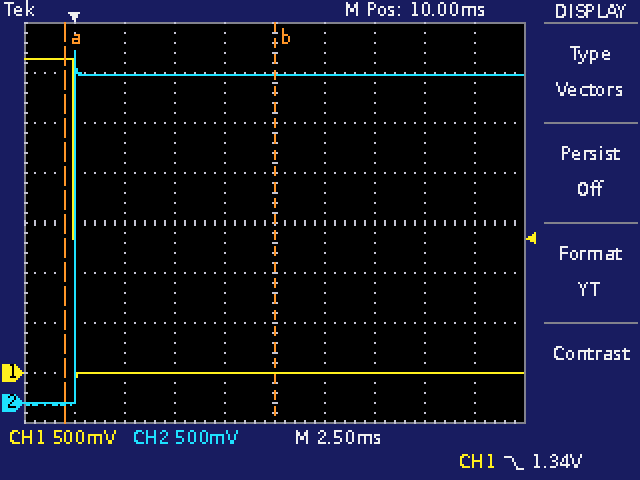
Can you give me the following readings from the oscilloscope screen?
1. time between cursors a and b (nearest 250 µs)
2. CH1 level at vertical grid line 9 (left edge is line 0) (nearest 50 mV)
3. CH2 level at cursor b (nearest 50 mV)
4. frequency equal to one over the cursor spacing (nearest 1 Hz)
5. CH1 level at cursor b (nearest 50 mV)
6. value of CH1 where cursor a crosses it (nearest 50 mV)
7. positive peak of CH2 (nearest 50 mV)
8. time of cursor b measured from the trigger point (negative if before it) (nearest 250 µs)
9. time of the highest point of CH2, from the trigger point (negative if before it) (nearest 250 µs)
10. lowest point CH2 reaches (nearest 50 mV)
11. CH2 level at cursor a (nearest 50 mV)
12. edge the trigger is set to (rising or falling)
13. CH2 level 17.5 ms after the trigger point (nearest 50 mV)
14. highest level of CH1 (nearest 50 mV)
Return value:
10.50 ms
0 mV
3.30 V
95 Hz
0 mV
3.15 V
3.50 V
+10.00 ms
0.00 ms
0 mV
0 mV
falling
3.30 V
3.15 V
